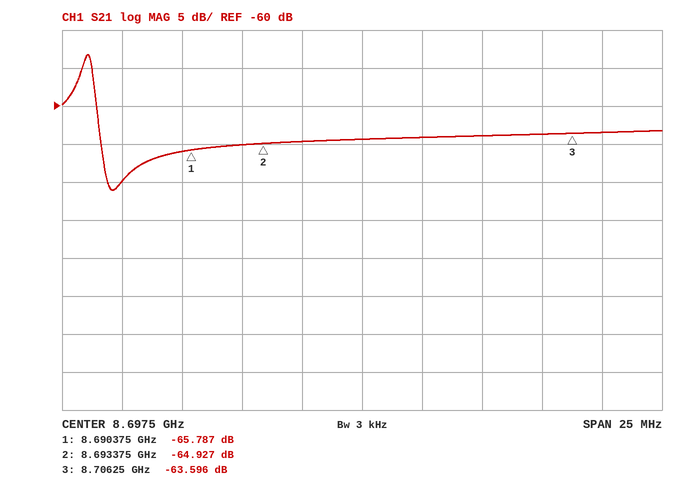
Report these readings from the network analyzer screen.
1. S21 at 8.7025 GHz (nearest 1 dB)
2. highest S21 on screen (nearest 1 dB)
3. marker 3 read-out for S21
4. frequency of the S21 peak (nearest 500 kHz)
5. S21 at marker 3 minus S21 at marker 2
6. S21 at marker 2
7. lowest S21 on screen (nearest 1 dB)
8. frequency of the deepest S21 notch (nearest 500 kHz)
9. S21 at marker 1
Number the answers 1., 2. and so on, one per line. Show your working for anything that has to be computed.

1. -64 dB
2. -53 dB
3. -63.596 dB
4. 8.6860 GHz
5. -63.596 − (-64.927) = 1.331 dB
6. -64.927 dB
7. -71 dB
8. 8.6870 GHz
9. -65.787 dB
